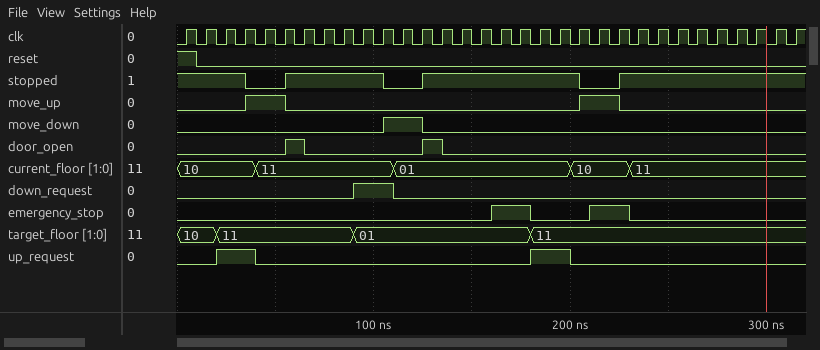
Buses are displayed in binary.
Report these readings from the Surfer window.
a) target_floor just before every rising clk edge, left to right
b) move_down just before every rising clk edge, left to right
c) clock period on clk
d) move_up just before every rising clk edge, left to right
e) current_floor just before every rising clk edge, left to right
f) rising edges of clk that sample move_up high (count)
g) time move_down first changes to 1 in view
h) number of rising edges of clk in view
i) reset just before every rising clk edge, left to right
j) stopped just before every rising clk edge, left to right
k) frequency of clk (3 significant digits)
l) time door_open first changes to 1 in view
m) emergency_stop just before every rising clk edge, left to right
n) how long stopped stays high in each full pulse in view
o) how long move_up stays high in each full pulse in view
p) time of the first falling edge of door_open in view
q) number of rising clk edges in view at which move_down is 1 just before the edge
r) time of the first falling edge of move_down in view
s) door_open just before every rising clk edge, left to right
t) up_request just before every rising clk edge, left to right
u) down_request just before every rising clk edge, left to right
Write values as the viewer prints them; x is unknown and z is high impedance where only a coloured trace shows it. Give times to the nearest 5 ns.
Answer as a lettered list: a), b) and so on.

a) 10, 10, 11, 11, 11, 11, 11, 11, 11, 01, 01, 01, 01, 01, 01, 01, 01, 01, 11, 11, 11, 11, 11, 11, 11, 11, 11, 11, 11, 11, 11, 11
b) 0 0 0 0 0 0 0 0 0 0 0 1 1 0 0 0 0 0 0 0 0 0 0 0 0 0 0 0 0 0 0 0
c) 10 ns
d) 0 0 0 0 1 1 0 0 0 0 0 0 0 0 0 0 0 0 0 0 0 1 1 0 0 0 0 0 0 0 0 0
e) 10, 10, 10, 10, 11, 11, 11, 11, 11, 11, 11, 01, 01, 01, 01, 01, 01, 01, 01, 01, 10, 10, 10, 11, 11, 11, 11, 11, 11, 11, 11, 11
f) 4
g) 105 ns
h) 32
i) 1 0 0 0 0 0 0 0 0 0 0 0 0 0 0 0 0 0 0 0 0 0 0 0 0 0 0 0 0 0 0 0
j) 1 1 1 1 0 0 1 1 1 1 1 0 0 1 1 1 1 1 1 1 1 0 0 1 1 1 1 1 1 1 1 1
k) 100 MHz
l) 55 ns
m) 0 0 0 0 0 0 0 0 0 0 0 0 0 0 0 0 1 1 0 0 0 1 1 0 0 0 0 0 0 0 0 0
n) 50 ns, 80 ns
o) 20 ns, 20 ns
p) 65 ns
q) 2
r) 125 ns
s) 0 0 0 0 0 0 1 0 0 0 0 0 0 1 0 0 0 0 0 0 0 0 0 0 0 0 0 0 0 0 0 0
t) 0 0 1 1 0 0 0 0 0 0 0 0 0 0 0 0 0 0 1 1 0 0 0 0 0 0 0 0 0 0 0 0
u) 0 0 0 0 0 0 0 0 0 1 1 0 0 0 0 0 0 0 0 0 0 0 0 0 0 0 0 0 0 0 0 0
